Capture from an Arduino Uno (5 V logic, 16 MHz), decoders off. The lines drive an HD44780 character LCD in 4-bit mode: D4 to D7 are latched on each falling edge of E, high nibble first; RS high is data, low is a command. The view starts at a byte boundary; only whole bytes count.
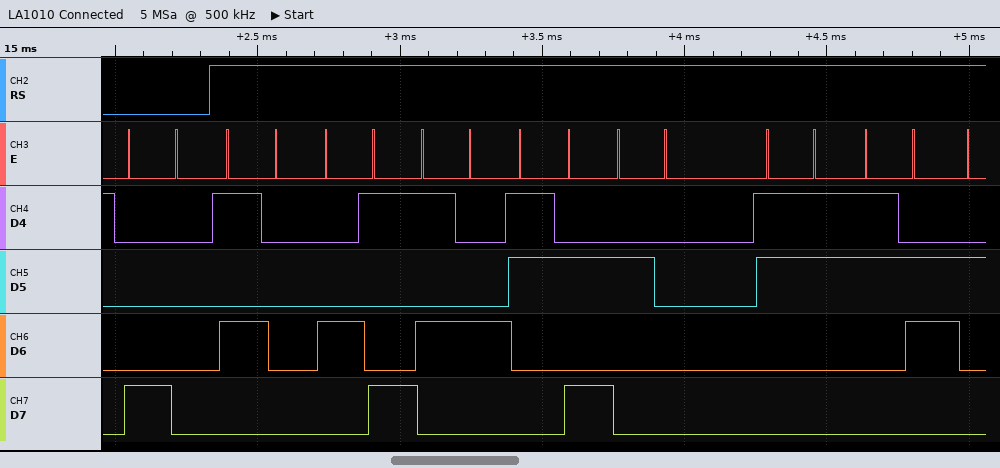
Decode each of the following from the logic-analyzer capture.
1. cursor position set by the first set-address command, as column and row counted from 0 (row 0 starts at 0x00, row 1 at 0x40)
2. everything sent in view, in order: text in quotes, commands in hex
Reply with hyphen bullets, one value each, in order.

- column 0, row 0
- 0x80 "PIT: 36"
